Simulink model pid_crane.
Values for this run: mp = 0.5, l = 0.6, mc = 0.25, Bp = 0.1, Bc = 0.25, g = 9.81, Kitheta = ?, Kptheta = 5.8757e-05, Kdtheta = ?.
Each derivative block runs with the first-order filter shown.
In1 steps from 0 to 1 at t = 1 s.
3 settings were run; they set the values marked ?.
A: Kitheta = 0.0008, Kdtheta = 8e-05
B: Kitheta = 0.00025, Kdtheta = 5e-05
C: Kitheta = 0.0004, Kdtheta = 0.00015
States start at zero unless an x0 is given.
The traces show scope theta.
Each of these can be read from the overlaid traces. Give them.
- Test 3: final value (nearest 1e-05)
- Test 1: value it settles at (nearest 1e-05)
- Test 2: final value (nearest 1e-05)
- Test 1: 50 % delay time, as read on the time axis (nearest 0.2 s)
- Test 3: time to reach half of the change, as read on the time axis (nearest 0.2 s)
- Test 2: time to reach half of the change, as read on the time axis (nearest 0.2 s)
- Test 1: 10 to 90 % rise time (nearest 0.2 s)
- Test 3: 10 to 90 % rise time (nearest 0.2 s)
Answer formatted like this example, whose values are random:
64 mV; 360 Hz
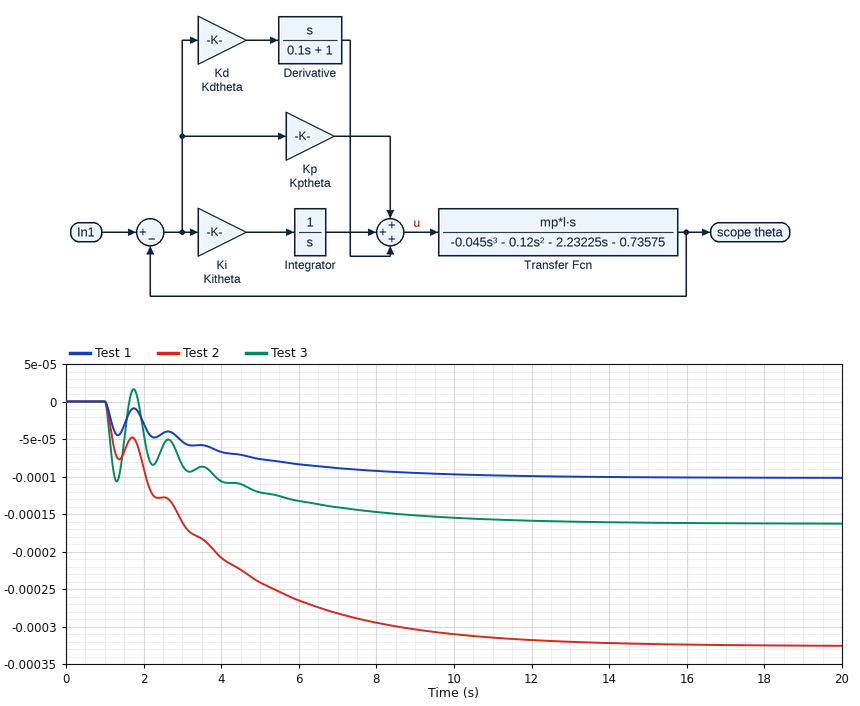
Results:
-0.00016; -0.00010; -0.00033; 3.0 s; 1.2 s; 3.0 s; 6.6 s; 6.8 s
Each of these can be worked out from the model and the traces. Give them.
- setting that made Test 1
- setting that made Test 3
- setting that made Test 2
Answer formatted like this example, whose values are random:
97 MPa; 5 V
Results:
B; C; A
